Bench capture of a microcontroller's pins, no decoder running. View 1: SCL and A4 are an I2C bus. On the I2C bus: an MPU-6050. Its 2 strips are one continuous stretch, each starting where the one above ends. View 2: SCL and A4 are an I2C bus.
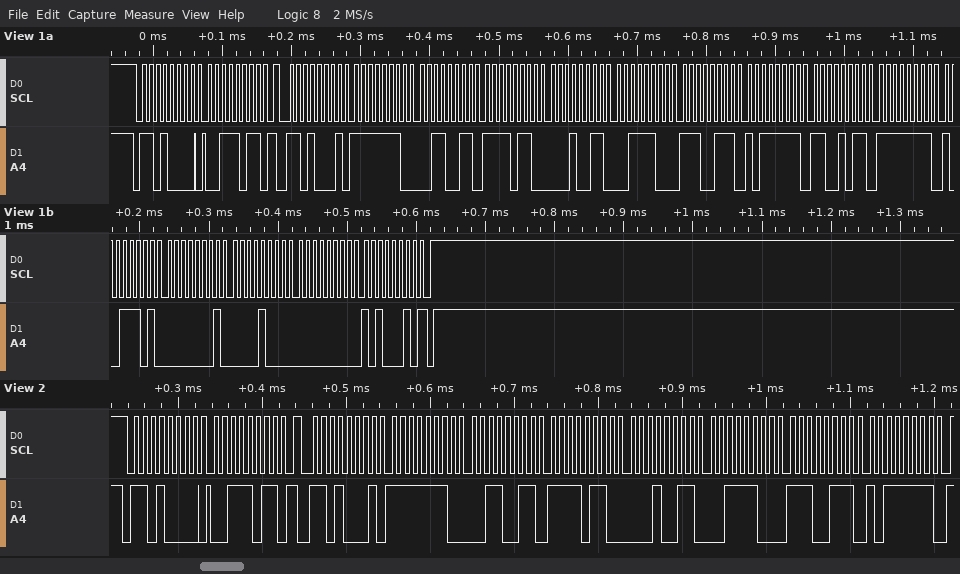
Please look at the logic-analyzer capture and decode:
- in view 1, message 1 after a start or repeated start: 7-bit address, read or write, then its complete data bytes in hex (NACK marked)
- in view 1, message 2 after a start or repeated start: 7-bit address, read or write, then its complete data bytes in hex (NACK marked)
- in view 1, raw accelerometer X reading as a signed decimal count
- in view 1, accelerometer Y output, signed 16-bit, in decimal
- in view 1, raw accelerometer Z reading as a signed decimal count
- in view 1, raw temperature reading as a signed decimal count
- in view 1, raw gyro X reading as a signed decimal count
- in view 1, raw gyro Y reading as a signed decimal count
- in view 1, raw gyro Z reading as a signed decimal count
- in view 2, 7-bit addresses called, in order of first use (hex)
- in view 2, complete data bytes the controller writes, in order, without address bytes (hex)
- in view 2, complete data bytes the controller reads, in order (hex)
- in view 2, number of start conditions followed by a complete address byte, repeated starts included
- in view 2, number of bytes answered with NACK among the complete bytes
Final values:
0x68 write: 3B
0x68 read: FE 33 F6 13 3C E7 BF CB FF 9D 01 08 00 A2 NACK
-461
-2541
15591
-16437
-99
264
162
0x68
3B
FE 33 F6 13 3C E7 BF
2
0
